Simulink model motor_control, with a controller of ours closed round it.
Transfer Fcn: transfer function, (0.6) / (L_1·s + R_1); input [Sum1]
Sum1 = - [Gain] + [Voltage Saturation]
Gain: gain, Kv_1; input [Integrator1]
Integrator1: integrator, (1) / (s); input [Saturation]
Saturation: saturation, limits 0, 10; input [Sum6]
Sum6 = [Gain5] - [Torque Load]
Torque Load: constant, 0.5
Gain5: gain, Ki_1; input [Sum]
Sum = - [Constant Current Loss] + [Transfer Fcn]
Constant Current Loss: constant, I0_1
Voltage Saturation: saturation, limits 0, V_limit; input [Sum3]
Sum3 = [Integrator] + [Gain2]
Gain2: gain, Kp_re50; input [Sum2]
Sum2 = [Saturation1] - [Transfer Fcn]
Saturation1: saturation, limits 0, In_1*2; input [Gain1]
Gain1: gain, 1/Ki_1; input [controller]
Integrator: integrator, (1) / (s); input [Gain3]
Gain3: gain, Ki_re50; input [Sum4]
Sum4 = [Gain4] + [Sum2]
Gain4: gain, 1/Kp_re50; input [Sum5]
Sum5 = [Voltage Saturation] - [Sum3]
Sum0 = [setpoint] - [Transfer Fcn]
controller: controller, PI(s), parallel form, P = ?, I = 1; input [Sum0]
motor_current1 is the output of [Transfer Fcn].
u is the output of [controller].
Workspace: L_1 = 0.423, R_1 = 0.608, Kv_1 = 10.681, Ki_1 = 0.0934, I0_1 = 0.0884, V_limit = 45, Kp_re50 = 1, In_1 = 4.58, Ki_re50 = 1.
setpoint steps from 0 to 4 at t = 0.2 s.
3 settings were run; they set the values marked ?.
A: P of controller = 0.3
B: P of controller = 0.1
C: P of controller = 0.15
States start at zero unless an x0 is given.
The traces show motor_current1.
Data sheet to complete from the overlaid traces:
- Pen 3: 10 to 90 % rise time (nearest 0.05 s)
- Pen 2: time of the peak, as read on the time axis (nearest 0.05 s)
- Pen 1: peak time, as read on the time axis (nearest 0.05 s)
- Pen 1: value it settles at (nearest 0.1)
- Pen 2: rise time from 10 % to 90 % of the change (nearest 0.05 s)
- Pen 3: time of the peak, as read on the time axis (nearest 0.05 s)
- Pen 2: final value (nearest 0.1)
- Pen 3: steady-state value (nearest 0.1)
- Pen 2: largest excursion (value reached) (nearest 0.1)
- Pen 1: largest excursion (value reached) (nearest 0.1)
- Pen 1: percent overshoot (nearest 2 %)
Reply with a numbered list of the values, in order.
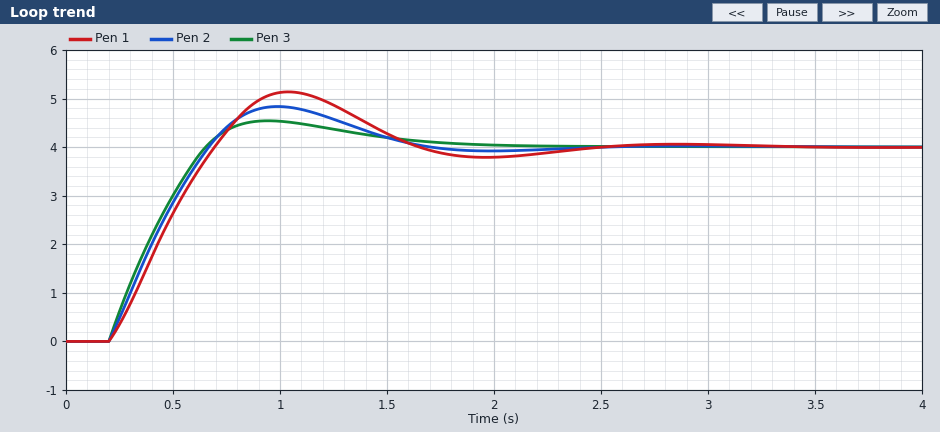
1. 0.35 s
2. 1.00 s
3. 1.05 s
4. 4.0
5. 0.35 s
6. 0.95 s
7. 4.0
8. 4.0
9. 4.8
10. 5.1
11. 28 %
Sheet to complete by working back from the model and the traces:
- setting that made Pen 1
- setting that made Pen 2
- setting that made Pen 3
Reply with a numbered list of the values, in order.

1. B
2. C
3. A
